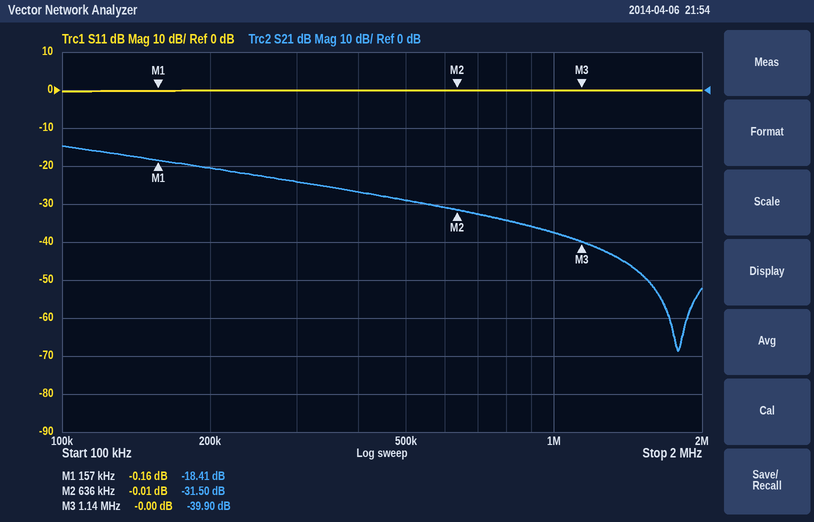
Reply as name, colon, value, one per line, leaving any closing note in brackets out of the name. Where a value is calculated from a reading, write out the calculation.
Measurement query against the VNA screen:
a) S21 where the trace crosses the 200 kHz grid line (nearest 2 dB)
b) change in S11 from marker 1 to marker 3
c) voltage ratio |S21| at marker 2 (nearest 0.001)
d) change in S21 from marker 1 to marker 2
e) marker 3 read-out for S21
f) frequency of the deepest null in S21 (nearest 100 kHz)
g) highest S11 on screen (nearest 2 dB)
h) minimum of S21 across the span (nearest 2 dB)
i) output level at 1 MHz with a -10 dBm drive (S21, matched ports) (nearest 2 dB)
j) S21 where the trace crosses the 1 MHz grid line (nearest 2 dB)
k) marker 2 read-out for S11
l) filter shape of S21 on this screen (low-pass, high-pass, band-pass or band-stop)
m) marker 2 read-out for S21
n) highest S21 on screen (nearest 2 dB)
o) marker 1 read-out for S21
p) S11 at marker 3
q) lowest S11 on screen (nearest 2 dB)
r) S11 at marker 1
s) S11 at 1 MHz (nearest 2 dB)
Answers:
S21 where the trace crosses the 200 kHz grid line: -20 dB
change in S11 from marker 1 to marker 3: -0 − (-0.16) = 0.16 dB
voltage ratio |S21| at marker 2: 10^(-31.5/20) ≈ 0.027
change in S21 from marker 1 to marker 2: -31.5 − (-18.41) = -13.09 dB
marker 3 read-out for S21: -39.90 dB
frequency of the deepest null in S21: 1.8 MHz
highest S11 on screen: 0 dB
minimum of S21 across the span: -68 dB
output level at 1 MHz with a -10 dBm drive (S21, matched ports): -10 dBm + (-38 dB) = -48 dBm
S21 where the trace crosses the 1 MHz grid line: -38 dB
marker 2 read-out for S11: -0.01 dB
filter shape of S21 on this screen: low-pass
marker 2 read-out for S21: -31.50 dB
highest S21 on screen: -14 dB
marker 1 read-out for S21: -18.41 dB
S11 at marker 3: -0.00 dB
lowest S11 on screen: 0 dB
S11 at marker 1: -0.16 dB
S11 at 1 MHz: 0 dB
